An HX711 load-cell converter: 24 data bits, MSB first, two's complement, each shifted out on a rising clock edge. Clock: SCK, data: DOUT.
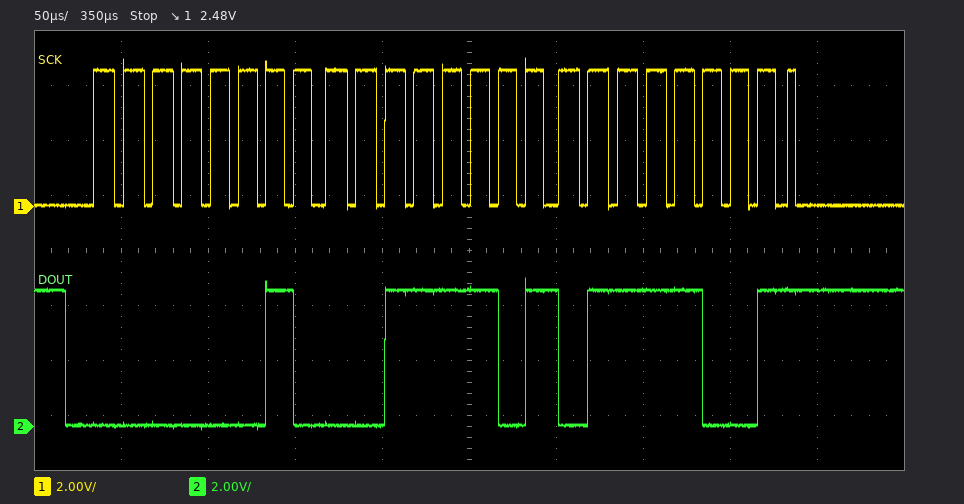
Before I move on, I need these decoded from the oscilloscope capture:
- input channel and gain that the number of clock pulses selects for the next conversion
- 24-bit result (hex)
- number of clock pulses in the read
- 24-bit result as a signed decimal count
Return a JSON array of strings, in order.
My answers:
["channel A, gain 128", "0x023D79", "25", "146809"]
